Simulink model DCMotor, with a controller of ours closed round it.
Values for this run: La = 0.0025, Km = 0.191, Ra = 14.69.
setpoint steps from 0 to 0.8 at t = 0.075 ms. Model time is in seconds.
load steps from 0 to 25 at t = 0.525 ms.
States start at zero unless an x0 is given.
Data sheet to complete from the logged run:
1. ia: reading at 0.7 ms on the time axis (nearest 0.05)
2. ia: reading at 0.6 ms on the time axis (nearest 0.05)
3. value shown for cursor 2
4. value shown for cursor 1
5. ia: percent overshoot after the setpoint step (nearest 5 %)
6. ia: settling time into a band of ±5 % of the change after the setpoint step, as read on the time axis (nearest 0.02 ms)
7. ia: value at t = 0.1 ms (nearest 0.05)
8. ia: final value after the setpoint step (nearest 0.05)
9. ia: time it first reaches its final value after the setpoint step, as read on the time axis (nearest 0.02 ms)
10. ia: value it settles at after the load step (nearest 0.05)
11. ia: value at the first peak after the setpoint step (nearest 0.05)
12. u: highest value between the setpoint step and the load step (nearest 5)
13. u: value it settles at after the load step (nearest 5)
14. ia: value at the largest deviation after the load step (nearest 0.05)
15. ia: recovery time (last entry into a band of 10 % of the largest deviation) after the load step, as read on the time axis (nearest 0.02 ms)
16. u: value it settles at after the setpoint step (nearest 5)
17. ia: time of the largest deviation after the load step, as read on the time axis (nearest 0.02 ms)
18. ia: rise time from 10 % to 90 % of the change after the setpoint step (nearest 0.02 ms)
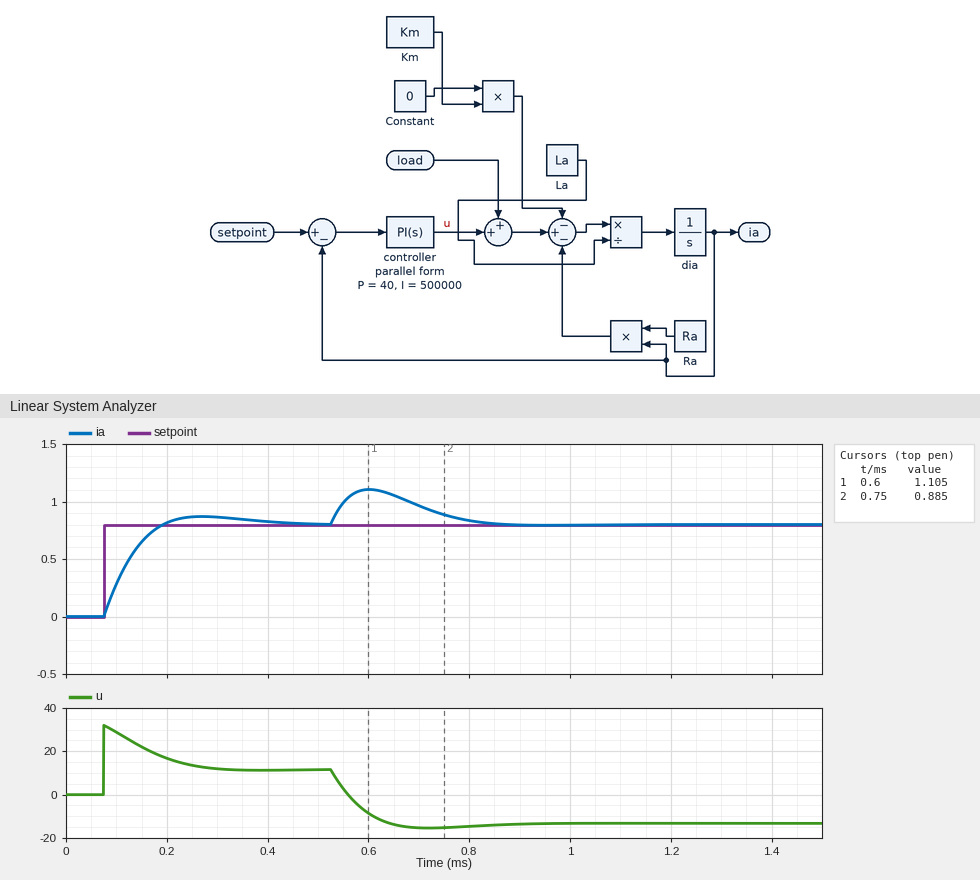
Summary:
0.95
1.10
0.885
1.105
10 %
0.36 ms
0.30
0.80
0.20 ms
0.80
0.85
30
-15
1.10
0.80 ms
10
0.60 ms
0.08 ms
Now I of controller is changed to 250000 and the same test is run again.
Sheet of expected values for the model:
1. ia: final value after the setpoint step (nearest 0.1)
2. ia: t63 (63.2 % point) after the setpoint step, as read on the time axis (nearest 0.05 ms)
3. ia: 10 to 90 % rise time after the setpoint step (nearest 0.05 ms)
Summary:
0.8
0.15 ms
0.15 ms
